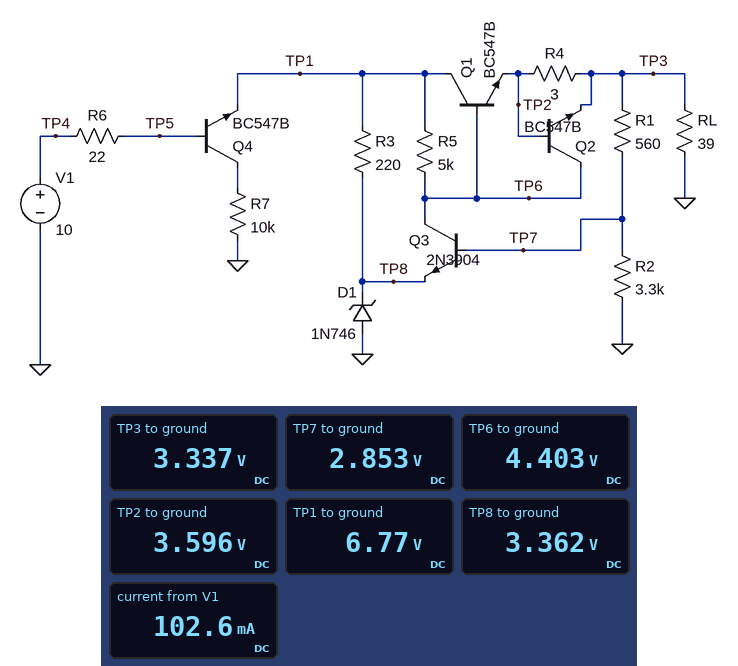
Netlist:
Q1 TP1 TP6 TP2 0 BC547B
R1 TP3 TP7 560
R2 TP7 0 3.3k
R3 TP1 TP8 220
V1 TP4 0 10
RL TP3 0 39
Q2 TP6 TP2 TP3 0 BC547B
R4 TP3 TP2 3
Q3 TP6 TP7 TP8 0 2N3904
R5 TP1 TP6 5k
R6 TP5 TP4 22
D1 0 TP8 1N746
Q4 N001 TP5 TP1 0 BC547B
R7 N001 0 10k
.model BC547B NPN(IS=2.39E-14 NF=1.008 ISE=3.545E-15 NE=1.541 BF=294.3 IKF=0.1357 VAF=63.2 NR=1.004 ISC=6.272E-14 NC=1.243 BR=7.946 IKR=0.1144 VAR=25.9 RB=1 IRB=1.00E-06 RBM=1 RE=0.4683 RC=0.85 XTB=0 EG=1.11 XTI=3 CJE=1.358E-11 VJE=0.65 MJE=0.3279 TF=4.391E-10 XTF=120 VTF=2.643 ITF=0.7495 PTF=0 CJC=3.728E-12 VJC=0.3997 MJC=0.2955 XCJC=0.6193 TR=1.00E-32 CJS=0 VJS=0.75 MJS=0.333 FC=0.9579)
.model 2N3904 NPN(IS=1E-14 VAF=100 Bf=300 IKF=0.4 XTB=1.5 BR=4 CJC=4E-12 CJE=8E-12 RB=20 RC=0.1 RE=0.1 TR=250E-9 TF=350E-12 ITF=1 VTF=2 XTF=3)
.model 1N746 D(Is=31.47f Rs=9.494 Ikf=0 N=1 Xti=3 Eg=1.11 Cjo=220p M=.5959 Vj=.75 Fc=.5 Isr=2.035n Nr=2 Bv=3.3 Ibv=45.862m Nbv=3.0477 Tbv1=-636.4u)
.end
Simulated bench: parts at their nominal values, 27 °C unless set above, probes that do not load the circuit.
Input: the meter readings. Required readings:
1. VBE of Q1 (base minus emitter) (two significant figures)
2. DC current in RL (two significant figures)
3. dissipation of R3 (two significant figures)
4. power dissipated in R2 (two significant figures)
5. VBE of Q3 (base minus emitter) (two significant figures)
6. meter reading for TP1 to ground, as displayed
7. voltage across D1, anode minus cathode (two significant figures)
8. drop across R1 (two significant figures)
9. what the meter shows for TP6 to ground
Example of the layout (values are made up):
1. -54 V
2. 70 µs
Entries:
1. 810 mV
2. 86 mA
3. 53 mW
4. 2.5 mW
5. -510 mV
6. 6.77 V
7. -3.4 V
8. 480 mV
9. 4.403 V
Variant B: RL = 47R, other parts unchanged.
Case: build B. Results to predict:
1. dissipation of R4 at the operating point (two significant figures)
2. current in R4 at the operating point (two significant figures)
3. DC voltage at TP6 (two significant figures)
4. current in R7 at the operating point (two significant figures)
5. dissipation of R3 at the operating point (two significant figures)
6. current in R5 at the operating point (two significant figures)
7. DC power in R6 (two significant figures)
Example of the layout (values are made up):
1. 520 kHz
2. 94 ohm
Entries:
1. 19 mW
2. 80 mA
3. 4.8 V
4. 700 µA
5. 57 mW
6. 430 µA
7. 210 mW
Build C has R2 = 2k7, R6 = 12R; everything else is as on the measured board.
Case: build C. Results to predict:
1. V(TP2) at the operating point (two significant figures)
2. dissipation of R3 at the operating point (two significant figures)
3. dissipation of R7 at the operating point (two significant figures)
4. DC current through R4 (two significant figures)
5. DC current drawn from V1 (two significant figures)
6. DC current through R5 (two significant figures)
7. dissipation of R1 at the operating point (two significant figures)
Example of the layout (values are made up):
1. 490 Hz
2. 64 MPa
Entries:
1. 4.0 V
2. 80 mW
3. 5.9 mW
4. 97 mA
5. 120 mA
6. 550 µA
7. 740 µW
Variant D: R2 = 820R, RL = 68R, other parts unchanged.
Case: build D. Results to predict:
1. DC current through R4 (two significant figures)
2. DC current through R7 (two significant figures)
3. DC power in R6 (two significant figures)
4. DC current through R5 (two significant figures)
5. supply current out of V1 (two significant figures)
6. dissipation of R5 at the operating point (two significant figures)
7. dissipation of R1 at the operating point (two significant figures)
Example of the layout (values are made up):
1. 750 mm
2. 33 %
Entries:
1. 68 mA
2. 720 µA
3. 160 mW
4. 350 µA
5. 86 mA
6. 610 µW
7. 5.8 mW
